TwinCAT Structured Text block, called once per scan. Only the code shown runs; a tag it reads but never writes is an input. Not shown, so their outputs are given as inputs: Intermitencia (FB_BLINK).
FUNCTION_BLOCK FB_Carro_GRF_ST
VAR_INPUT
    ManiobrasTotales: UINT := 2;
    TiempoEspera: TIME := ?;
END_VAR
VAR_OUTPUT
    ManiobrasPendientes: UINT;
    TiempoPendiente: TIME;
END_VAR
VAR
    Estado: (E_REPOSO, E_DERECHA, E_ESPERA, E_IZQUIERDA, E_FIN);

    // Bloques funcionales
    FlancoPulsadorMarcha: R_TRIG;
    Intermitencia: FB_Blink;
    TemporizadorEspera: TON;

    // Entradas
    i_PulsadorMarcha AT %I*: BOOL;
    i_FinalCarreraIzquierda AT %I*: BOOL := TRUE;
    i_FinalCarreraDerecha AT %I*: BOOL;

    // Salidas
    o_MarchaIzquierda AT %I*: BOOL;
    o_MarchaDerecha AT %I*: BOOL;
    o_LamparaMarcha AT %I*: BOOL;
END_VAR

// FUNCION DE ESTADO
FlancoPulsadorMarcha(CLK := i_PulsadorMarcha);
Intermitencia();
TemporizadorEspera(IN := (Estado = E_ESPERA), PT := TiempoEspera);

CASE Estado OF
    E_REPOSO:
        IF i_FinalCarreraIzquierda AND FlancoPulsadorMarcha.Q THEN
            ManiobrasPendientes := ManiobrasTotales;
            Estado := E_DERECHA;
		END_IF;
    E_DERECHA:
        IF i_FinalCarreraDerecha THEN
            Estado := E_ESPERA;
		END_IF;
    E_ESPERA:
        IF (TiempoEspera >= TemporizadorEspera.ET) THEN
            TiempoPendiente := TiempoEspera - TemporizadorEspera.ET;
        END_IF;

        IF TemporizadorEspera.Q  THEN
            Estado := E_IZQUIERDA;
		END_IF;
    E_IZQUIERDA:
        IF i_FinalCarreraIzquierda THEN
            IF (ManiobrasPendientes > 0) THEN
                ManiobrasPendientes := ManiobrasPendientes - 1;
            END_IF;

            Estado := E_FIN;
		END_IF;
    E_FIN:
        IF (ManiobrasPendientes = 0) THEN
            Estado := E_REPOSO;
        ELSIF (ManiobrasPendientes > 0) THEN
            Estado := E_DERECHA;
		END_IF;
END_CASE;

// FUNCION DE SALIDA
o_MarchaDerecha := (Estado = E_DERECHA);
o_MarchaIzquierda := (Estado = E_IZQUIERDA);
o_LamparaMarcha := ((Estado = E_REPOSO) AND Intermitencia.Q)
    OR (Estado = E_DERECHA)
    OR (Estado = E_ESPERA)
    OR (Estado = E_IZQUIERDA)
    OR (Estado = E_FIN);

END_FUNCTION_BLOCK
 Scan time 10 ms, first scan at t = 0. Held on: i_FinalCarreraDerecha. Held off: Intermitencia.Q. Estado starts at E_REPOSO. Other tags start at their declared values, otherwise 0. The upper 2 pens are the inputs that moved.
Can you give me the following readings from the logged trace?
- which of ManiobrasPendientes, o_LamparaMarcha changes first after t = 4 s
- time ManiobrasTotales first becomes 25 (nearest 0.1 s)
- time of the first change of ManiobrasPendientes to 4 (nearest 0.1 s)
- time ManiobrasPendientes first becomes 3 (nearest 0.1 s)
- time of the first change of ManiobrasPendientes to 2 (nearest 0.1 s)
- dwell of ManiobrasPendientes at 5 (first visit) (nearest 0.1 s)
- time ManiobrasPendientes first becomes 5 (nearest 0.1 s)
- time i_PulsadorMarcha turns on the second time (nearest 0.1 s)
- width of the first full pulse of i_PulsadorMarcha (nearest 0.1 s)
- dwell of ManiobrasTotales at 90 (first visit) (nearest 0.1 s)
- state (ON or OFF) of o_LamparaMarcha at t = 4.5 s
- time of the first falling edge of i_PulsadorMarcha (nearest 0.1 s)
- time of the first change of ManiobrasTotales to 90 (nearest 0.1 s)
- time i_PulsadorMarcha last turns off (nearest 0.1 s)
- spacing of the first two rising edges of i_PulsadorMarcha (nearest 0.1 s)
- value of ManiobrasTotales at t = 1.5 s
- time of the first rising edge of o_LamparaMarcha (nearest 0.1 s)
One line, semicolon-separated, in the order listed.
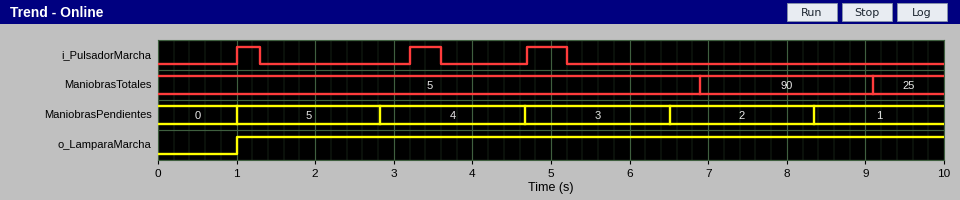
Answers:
ManiobrasPendientes; 9.1 s; 2.8 s; 4.7 s; 6.5 s; 1.8 s; 1.0 s; 3.2 s; 0.3 s; 2.2 s; ON; 1.3 s; 6.9 s; 5.2 s; 2.2 s; 5; 1.0 s
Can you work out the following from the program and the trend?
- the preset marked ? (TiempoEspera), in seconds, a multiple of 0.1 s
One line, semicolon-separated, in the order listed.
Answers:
1.8 s
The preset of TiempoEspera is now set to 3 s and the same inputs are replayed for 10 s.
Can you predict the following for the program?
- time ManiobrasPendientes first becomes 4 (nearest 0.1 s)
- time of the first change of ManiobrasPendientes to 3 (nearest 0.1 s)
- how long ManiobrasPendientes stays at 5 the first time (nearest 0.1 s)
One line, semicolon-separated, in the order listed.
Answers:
4.0 s; 7.1 s; 3.0 s
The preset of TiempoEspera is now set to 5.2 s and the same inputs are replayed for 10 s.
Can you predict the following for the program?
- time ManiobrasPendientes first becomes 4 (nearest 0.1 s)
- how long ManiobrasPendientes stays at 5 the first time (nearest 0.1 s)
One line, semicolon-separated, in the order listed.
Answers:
6.2 s; 5.2 s
